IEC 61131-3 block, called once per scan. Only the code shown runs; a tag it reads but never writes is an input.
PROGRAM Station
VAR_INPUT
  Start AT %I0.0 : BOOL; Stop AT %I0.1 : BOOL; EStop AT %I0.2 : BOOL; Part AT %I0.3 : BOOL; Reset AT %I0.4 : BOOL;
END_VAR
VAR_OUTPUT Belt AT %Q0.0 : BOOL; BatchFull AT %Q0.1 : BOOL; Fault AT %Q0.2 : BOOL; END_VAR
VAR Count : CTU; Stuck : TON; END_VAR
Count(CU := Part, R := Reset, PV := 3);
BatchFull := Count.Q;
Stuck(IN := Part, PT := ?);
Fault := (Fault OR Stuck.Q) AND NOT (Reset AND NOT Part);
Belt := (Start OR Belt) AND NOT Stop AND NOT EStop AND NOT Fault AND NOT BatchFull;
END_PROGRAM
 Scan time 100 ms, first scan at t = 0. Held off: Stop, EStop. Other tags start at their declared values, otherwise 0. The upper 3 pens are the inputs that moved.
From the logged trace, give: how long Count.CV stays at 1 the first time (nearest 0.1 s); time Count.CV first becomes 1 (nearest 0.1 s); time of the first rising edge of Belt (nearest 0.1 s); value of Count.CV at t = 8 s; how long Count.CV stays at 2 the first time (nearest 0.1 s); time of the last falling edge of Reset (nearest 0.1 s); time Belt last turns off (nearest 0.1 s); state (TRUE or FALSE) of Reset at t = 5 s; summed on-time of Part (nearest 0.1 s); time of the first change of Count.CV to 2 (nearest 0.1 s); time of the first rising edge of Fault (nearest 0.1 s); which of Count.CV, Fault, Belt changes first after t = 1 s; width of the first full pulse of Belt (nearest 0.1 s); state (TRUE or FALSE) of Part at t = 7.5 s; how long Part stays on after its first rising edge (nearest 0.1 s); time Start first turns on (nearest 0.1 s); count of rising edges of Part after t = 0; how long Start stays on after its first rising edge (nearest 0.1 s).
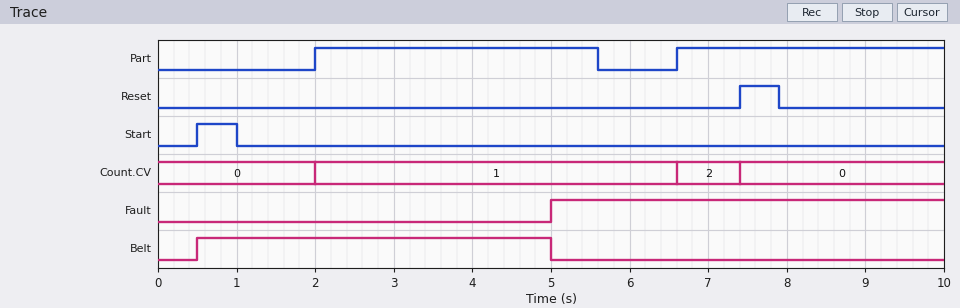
4.6 s
2.0 s
0.5 s
0
0.8 s
7.9 s
5.0 s
FALSE
7.0 s
6.6 s
5.0 s
Count.CV
4.5 s
TRUE
3.6 s
0.5 s
2
0.5 s
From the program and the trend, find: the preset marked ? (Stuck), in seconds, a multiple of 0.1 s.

3.0 s
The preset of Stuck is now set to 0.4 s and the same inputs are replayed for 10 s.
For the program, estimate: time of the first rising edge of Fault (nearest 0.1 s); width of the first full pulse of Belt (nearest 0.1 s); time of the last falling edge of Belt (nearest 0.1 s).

2.4 s
1.9 s
2.4 s
